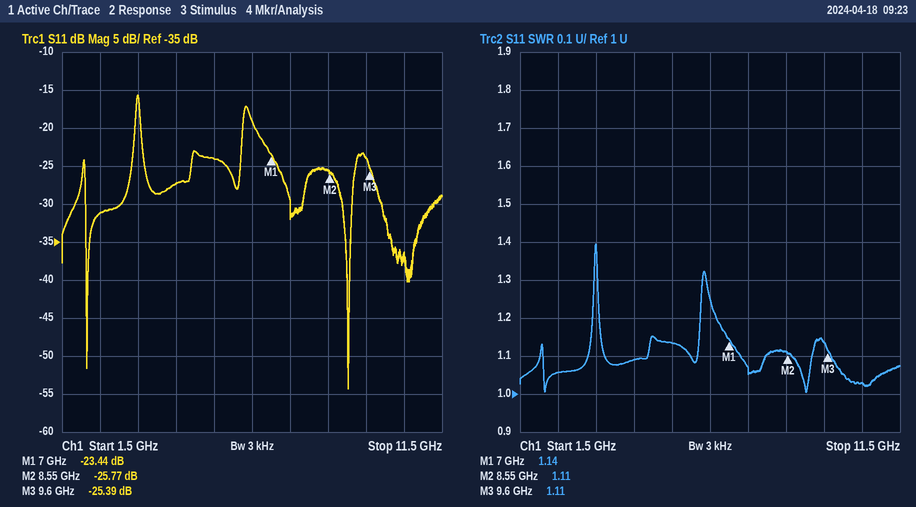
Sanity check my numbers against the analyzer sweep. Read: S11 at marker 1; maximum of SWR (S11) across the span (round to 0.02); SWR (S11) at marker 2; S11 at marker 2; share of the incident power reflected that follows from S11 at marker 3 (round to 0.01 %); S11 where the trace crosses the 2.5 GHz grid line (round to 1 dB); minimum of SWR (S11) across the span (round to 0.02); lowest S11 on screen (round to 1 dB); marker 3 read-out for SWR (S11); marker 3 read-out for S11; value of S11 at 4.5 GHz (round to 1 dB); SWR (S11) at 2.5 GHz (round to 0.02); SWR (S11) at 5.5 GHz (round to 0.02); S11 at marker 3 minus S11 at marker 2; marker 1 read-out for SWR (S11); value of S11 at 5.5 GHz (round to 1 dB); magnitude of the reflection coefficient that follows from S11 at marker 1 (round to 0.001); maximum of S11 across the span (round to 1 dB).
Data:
-23.44 dB
1.40
1.11
-25.77 dB
0.29 %
-31 dB
1.00
-54 dB
1.11
-25.39 dB
-27 dB
1.06
1.14
0.38 dB
1.14
-24 dB
0.067
-16 dB
